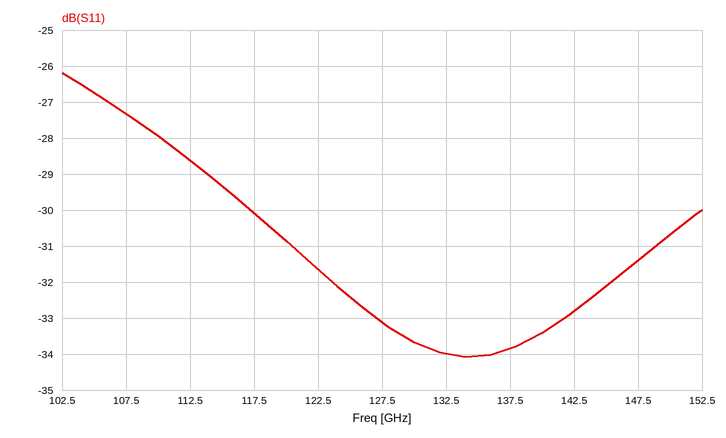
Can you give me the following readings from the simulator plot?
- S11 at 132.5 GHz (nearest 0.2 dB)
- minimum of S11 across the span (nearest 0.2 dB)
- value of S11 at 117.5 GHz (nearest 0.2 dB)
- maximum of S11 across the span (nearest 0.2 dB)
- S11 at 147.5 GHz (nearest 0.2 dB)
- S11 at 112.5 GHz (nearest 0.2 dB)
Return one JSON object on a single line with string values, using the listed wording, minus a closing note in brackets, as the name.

{"S11 at 132.5 GHz": "-34.0 dB", "minimum of S11 across the span": "-34.0 dB", "value of S11 at 117.5 GHz": "-30.0 dB", "maximum of S11 across the span": "-26.2 dB", "S11 at 147.5 GHz": "-31.4 dB", "S11 at 112.5 GHz": "-28.6 dB"}
